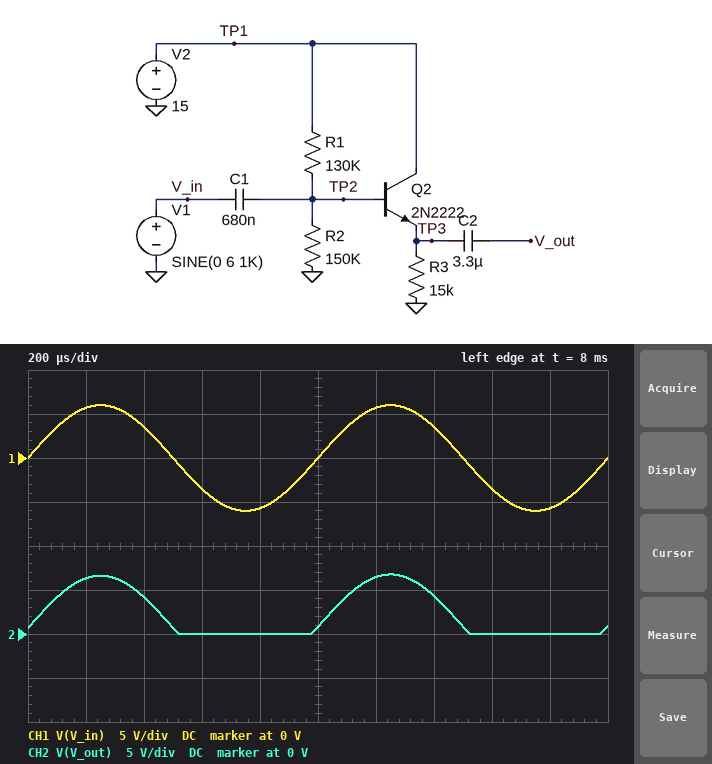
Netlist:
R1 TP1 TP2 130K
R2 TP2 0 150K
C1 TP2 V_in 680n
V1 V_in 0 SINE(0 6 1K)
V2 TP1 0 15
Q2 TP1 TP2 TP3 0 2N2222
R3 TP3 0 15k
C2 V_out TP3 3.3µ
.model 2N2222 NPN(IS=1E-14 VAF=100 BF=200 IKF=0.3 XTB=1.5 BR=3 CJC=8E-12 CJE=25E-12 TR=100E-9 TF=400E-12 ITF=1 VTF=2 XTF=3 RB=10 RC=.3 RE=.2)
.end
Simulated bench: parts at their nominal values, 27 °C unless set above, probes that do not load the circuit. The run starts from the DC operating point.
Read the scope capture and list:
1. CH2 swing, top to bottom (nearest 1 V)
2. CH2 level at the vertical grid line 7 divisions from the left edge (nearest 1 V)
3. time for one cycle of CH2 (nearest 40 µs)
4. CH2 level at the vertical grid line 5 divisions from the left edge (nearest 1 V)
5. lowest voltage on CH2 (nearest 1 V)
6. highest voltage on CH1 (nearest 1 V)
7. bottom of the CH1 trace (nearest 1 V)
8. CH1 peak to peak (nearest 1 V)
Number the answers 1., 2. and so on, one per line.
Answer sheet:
1. 7 V
2. 4 V
3. 1.00 ms
4. 1 V
5. 0 V
6. 6 V
7. -6 V
8. 12 V
